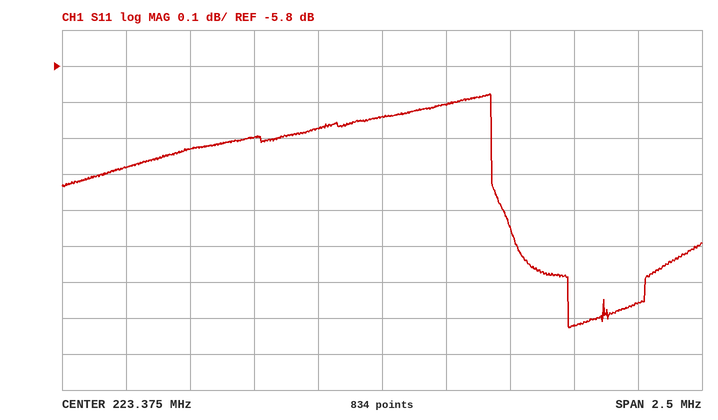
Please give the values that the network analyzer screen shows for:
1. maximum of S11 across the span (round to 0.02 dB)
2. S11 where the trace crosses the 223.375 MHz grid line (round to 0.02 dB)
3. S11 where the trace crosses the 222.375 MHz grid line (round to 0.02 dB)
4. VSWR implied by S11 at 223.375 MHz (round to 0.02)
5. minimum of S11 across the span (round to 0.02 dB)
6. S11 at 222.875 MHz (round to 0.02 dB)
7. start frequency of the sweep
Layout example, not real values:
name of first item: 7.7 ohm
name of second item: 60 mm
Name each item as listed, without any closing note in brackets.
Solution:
maximum of S11 across the span: -5.88 dB
S11 where the trace crosses the 223.375 MHz grid line: -5.94 dB
S11 where the trace crosses the 222.375 MHz grid line: -6.08 dB
VSWR implied by S11 at 223.375 MHz: 3.04
minimum of S11 across the span: -6.52 dB
S11 at 222.875 MHz: -6.00 dB
start frequency of the sweep: 222.125 MHz
